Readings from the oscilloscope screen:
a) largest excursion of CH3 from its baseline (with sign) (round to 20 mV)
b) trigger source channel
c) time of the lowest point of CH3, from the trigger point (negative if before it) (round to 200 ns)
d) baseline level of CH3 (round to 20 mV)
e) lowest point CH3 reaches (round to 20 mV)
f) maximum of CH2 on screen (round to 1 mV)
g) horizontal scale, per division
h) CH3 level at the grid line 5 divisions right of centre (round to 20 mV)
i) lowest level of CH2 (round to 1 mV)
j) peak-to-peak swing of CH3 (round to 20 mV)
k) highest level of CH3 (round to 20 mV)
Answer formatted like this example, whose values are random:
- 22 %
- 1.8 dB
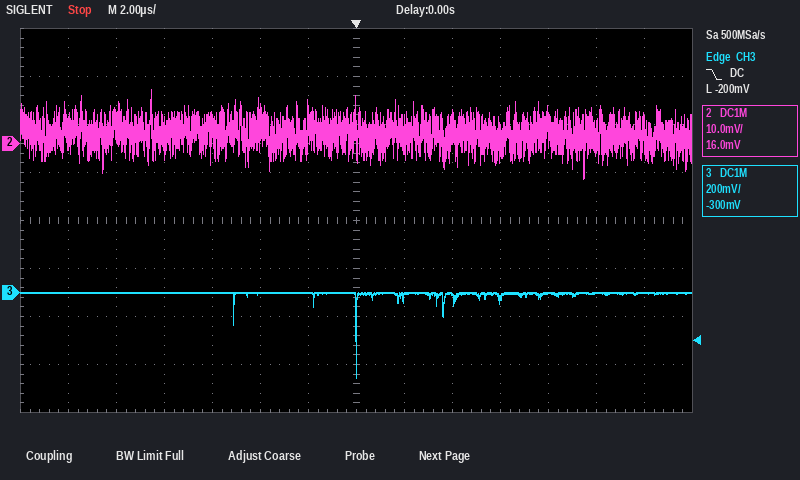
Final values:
- -360 mV
- CH3
- 0.0 µs
- 0 mV
- -360 mV
- 11 mV
- 2 µs
- 0 mV
- -7 mV
- 360 mV
- 0 mV
